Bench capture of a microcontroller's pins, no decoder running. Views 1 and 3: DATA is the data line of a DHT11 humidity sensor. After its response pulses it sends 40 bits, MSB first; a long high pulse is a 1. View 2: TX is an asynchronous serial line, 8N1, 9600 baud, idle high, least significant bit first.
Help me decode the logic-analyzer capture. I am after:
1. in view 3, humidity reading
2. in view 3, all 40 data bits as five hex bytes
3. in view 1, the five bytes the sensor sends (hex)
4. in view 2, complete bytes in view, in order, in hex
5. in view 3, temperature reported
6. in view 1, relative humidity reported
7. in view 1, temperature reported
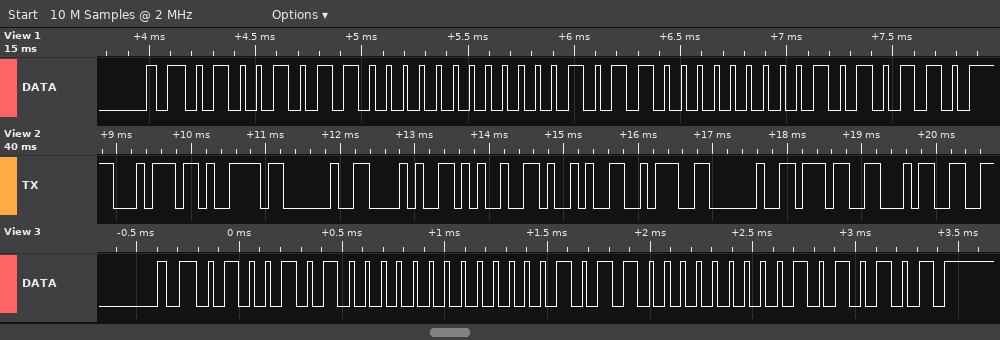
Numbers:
74 %
4A 00 0B 00 55
4B 00 0B 00 56
74 79 20 28 25 29 3A 20 37 34
11.0 °C
75 %
11.0 °C
